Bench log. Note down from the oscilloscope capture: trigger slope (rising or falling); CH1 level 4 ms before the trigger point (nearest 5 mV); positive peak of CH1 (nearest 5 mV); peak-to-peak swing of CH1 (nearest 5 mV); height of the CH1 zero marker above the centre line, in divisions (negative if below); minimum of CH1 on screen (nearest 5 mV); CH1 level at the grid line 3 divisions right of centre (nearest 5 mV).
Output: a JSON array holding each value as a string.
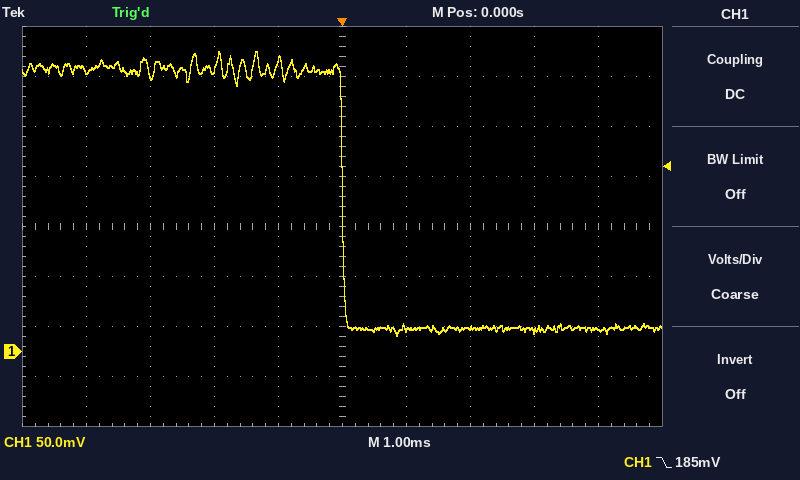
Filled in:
["falling", "280 mV", "300 mV", "285 mV", "-2.5 div", "15 mV", "20 mV"]
